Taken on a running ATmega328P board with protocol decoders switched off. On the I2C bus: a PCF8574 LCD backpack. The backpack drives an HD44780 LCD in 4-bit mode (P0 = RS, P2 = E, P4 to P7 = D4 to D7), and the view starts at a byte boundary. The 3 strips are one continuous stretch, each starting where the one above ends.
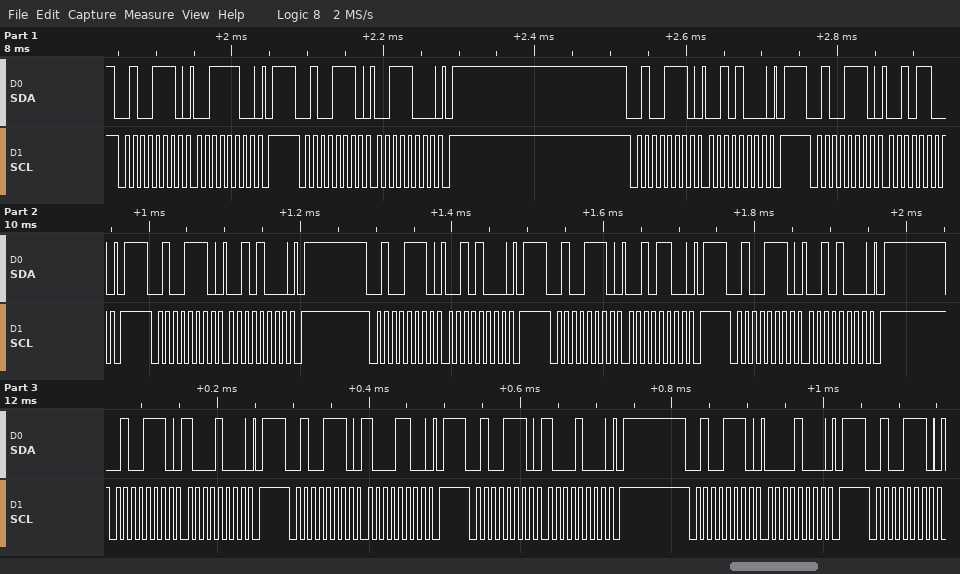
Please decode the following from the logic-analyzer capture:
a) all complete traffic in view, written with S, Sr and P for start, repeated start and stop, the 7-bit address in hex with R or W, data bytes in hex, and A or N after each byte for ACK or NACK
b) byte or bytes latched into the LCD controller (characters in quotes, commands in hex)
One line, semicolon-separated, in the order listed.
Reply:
S 27W A 3C A P S 27W A 38 A P S 27W A 28 A P S 27W A 2C A P S 27W A 28 A P S 27W A 28 A P S 27W A 2C A P S 27W A 28 A P S 27W A 88 A P S 27W A 8C A P S 27W A 88 A P S 27W A 08 A P S 27W A; 0x28
